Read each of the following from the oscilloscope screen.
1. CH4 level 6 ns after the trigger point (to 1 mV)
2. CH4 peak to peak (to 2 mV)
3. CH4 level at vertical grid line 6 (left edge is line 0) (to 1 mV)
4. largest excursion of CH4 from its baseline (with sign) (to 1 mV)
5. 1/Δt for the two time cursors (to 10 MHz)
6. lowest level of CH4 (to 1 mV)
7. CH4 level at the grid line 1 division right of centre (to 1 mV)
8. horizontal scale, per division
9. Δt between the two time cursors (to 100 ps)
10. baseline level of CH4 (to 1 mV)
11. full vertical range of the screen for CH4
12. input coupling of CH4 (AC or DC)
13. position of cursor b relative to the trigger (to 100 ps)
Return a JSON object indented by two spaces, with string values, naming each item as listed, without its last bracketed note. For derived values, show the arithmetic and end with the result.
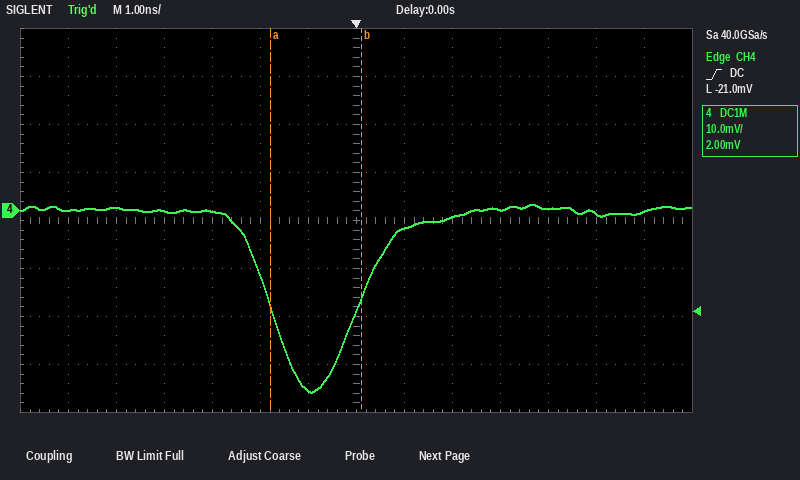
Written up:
{
  "CH4 level 6 ns after the trigger point": "0 mV",
  "CH4 peak to peak": "40 mV",
  "CH4 level at vertical grid line 6 (left edge is line 0)": "-37 mV",
  "largest excursion of CH4 from its baseline (with sign)": "-38 mV − (0 mV) = -38 mV",
  "1/Δt for the two time cursors": "1 / 1.9 ns ≈ 530 MHz",
  "lowest level of CH4": "-38 mV",
  "CH4 level at the grid line 1 division right of centre": "-4 mV",
  "horizontal scale, per division": "1 ns",
  "Δt between the two time cursors": "1.9 ns",
  "baseline level of CH4": "0 mV",
  "full vertical range of the screen for CH4": "80 mV",
  "input coupling of CH4": "DC",
  "position of cursor b relative to the trigger": "+100 ps"
}
